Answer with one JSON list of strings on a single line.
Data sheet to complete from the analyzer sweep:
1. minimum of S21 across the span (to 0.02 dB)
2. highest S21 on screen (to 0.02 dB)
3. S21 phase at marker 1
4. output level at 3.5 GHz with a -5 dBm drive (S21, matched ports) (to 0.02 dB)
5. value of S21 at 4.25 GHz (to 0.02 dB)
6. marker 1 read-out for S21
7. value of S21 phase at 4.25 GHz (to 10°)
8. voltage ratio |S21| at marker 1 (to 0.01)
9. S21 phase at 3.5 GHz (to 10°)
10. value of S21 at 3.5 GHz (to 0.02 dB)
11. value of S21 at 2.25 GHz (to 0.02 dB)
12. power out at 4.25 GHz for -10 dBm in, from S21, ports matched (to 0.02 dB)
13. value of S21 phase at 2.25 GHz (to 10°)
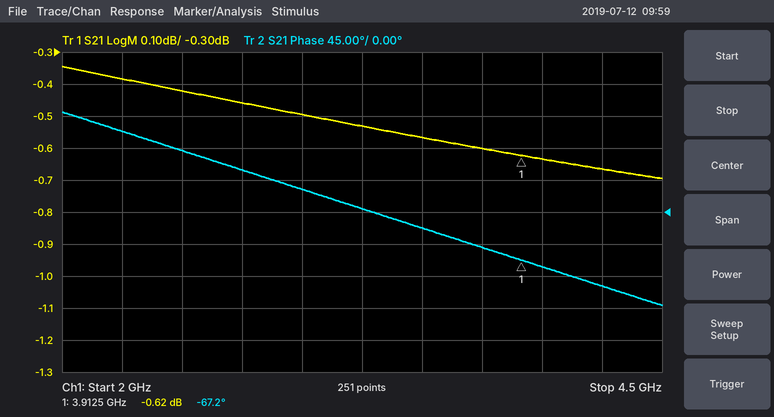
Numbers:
["-0.70 dB", "-0.34 dB", "-67.2°", "-5.56 dBm", "-0.66 dB", "-0.62 dB", "-100°", "0.93", "-20°", "-0.56 dB", "-0.38 dB", "-10.66 dBm", "110°"]
